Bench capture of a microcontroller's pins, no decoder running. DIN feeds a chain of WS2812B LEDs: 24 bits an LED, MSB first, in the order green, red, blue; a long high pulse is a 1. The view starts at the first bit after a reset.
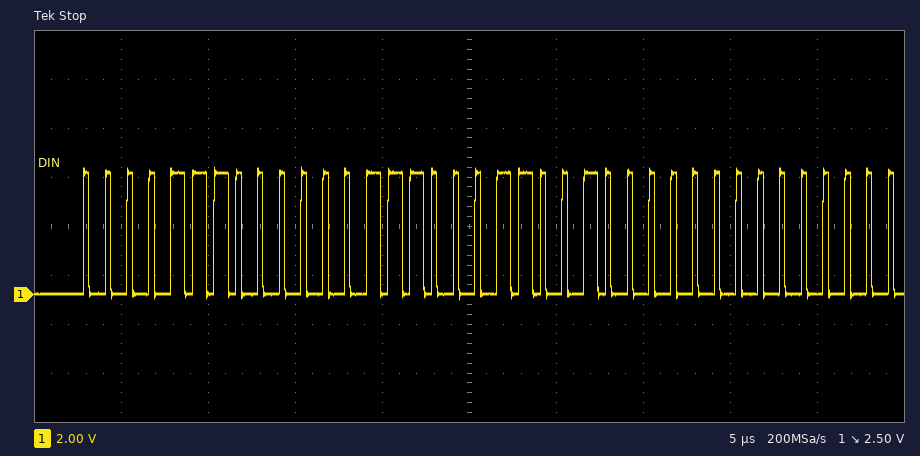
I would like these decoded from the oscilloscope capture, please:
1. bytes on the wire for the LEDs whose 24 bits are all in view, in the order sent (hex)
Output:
0E 07 19
